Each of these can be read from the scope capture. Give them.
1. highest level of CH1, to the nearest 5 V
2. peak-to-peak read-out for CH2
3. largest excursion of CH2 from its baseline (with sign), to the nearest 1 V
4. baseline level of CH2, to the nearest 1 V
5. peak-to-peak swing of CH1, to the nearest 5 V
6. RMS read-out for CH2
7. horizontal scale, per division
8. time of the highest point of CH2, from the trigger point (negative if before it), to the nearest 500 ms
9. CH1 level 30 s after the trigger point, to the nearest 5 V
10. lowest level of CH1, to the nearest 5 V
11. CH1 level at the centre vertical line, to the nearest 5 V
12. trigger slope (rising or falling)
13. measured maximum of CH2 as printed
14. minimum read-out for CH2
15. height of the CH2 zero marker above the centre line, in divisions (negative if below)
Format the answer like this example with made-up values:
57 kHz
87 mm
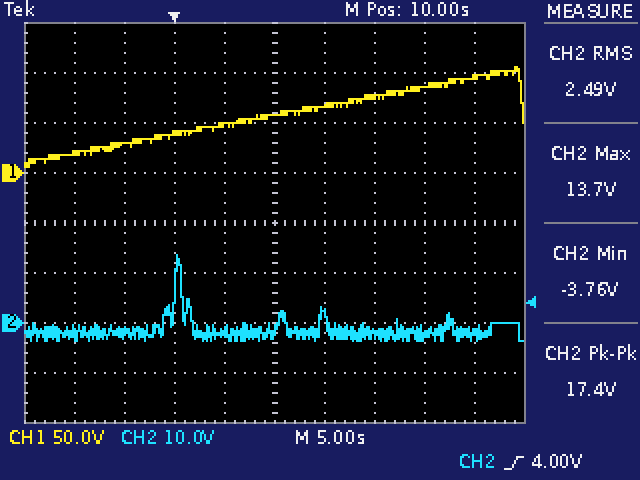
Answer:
105 V
17.4 V
+16 V
-2 V
100 V
2.49 V
5 s
+500 ms
95 V
5 V
60 V
rising
13.7 V
-3.76 V
-2.0 div
